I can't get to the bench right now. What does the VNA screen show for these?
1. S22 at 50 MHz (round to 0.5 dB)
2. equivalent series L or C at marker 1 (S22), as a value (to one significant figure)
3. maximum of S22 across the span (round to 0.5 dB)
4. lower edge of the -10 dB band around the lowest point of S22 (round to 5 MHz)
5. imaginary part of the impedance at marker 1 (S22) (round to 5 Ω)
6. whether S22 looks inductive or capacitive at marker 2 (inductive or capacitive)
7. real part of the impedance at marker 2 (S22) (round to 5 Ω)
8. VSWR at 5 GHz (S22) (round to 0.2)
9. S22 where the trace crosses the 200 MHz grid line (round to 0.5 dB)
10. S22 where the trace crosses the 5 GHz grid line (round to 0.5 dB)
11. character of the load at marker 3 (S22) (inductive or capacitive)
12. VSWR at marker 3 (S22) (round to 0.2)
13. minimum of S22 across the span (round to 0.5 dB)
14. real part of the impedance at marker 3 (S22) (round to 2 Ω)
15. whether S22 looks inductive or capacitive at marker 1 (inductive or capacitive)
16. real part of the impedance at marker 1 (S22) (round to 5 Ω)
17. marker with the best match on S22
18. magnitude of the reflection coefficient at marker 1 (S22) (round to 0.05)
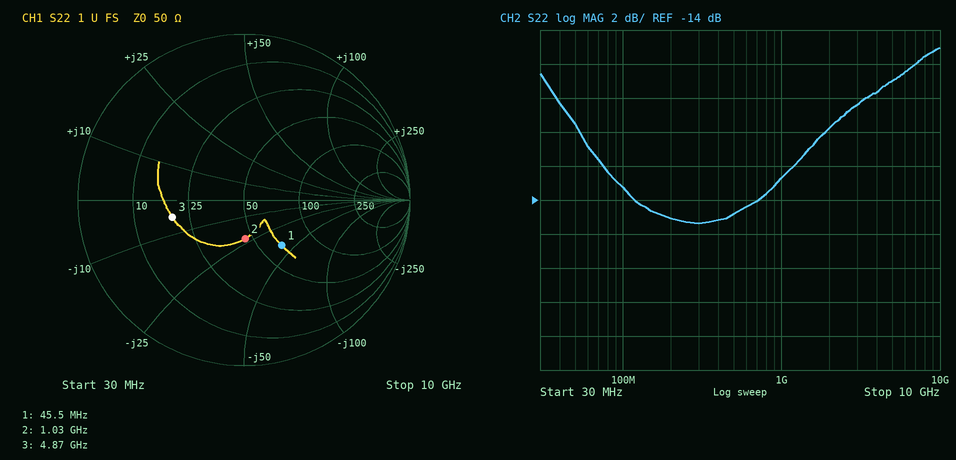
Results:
-9.5 dB
90 pF
-5.0 dB
55 MHz
-40 Ω
capacitive
45 Ω
2.6
-15.0 dB
-7.0 dB
capacitive
2.6
-15.5 dB
20 Ω
capacitive
65 Ω
marker 2
0.35
